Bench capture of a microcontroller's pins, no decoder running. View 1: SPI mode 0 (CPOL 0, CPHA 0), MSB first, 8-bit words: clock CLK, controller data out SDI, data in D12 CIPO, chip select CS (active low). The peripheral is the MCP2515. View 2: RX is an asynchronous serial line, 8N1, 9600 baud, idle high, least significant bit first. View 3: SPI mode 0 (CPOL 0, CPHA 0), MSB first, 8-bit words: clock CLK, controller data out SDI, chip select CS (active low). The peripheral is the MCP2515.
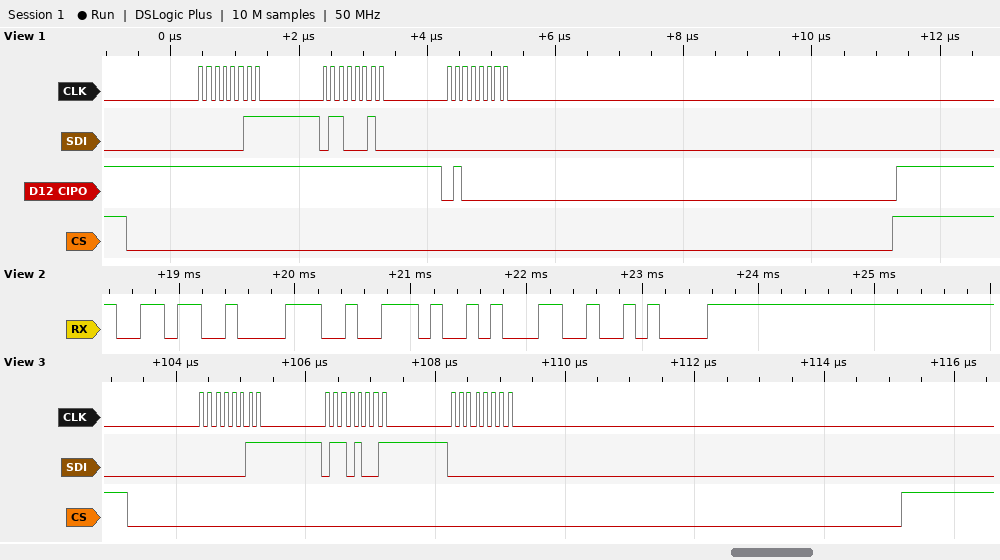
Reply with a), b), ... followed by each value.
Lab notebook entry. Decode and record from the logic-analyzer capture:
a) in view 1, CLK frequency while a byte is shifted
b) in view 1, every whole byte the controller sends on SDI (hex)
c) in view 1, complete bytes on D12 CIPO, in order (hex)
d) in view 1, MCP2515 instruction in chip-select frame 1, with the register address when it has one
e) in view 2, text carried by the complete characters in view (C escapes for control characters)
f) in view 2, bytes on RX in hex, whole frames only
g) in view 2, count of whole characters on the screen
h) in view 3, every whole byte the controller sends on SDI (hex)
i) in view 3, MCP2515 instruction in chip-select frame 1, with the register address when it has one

a) 8 MHz
b) 03 62 00
c) FF FF 40
d) READ 0x62
e) "68.1\n"
f) 36 38 2E 31 0A
g) 5
h) 03 69 00
i) READ 0x69
